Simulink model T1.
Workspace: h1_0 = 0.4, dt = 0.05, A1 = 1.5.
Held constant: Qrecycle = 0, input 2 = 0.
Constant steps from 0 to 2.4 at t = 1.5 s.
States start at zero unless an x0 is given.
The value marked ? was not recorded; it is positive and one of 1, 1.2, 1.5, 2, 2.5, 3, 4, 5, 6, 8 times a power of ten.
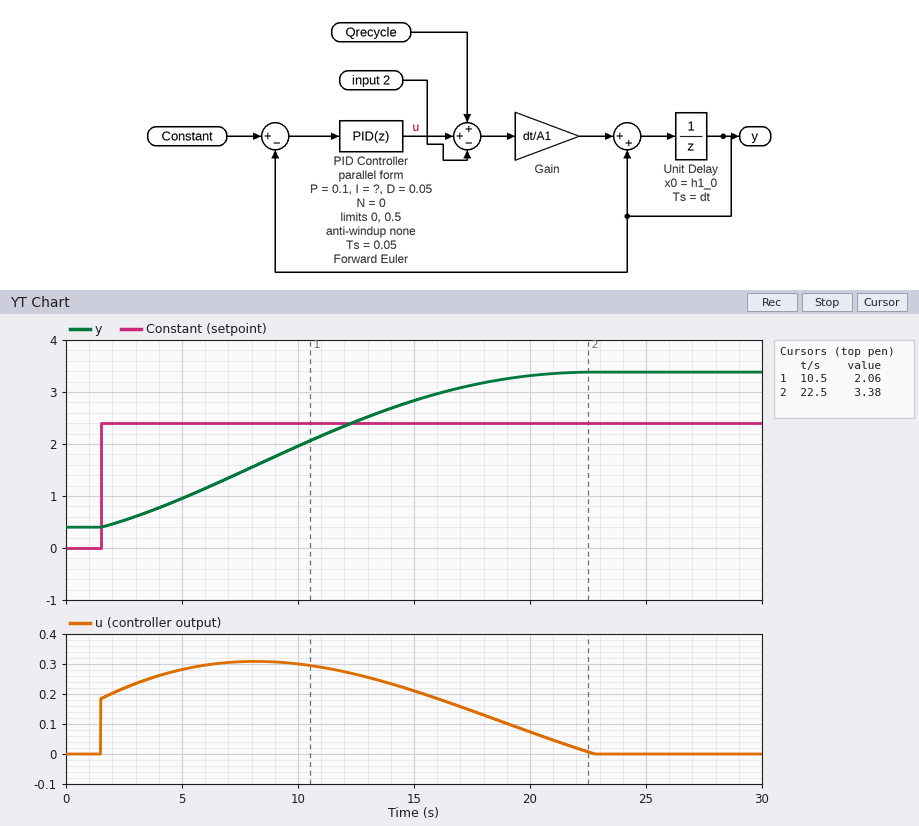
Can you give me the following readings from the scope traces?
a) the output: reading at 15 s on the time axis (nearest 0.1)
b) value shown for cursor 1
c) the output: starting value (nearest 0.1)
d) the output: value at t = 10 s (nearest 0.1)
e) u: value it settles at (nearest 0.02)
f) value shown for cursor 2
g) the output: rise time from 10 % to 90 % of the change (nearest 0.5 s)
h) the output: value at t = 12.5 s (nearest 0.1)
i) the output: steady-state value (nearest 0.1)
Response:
2.8
2.06
0.4
2.0
0.00
3.38
13.5 s
2.4
3.4
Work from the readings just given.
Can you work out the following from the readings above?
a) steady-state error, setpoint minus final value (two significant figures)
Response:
-1.0
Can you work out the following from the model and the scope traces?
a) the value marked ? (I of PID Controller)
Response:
0.025
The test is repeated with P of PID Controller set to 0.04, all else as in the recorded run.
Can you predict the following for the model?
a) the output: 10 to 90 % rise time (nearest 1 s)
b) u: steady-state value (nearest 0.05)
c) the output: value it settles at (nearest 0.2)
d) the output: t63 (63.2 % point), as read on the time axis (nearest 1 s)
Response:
14 s
0.00
3.8
14 s
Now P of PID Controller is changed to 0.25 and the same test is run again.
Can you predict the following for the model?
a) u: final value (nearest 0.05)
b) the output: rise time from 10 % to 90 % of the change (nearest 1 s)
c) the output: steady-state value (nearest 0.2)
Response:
0.00
10 s
2.8
